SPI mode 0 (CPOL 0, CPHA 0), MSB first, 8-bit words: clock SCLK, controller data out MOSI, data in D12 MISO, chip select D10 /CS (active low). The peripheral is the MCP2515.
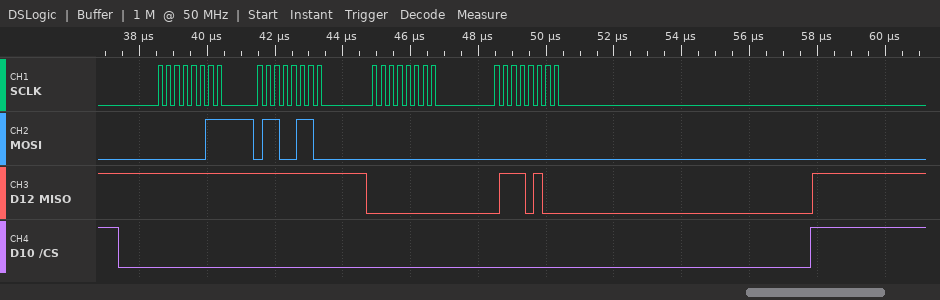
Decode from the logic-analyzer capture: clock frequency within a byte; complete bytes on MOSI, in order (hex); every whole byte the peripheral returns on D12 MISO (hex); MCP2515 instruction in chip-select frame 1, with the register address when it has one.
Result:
4 MHz
03 66 00 00
FF FF 00 74
READ 0x66
